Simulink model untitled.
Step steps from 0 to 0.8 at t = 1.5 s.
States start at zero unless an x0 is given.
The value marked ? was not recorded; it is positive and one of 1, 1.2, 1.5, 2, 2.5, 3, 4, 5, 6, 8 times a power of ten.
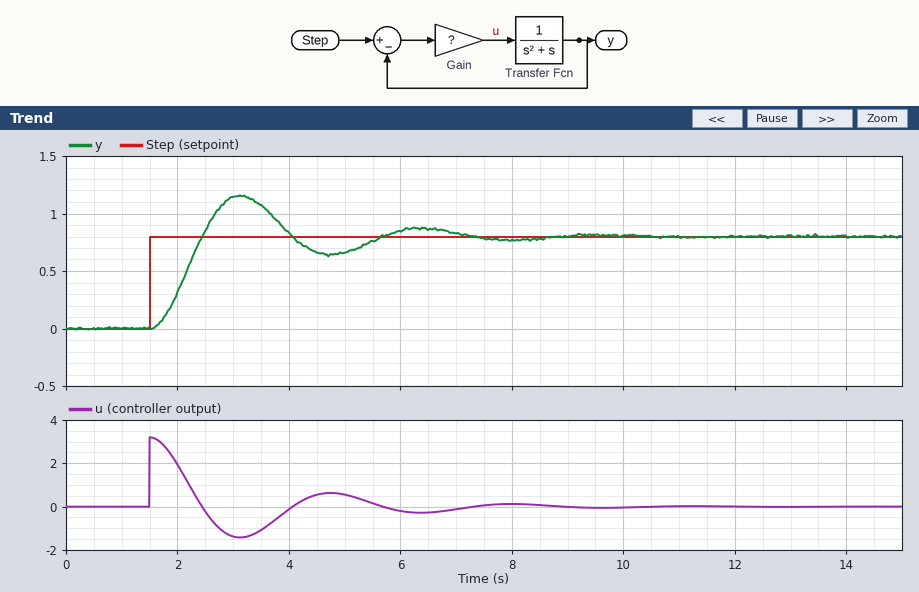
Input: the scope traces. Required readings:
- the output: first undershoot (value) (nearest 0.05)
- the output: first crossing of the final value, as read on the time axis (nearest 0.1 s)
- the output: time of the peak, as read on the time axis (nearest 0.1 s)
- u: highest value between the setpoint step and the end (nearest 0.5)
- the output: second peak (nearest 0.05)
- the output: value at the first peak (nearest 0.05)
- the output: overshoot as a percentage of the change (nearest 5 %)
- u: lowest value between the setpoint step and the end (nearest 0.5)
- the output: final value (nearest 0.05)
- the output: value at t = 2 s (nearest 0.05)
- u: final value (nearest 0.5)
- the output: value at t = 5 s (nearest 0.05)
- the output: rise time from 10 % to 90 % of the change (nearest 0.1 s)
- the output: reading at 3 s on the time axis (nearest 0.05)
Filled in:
0.65
2.4 s
3.1 s
3.0
0.85
1.15
45 %
-1.5
0.80
0.30
0.0
0.65
0.6 s
1.15
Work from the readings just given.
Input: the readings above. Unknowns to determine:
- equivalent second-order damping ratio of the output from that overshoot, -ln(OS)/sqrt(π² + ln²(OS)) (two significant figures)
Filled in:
0.25
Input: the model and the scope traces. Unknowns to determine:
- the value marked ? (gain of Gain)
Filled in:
4
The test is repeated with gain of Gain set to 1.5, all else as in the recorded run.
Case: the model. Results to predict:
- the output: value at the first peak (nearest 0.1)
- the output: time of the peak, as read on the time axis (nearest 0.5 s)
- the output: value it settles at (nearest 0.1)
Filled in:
1.0
4.5 s
0.8
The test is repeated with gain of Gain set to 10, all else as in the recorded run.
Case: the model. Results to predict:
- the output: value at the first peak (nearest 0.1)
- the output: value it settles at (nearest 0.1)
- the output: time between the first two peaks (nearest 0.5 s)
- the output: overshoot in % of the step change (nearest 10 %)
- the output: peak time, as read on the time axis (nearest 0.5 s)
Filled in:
1.3
0.8
2.0 s
60 %
2.5 s
